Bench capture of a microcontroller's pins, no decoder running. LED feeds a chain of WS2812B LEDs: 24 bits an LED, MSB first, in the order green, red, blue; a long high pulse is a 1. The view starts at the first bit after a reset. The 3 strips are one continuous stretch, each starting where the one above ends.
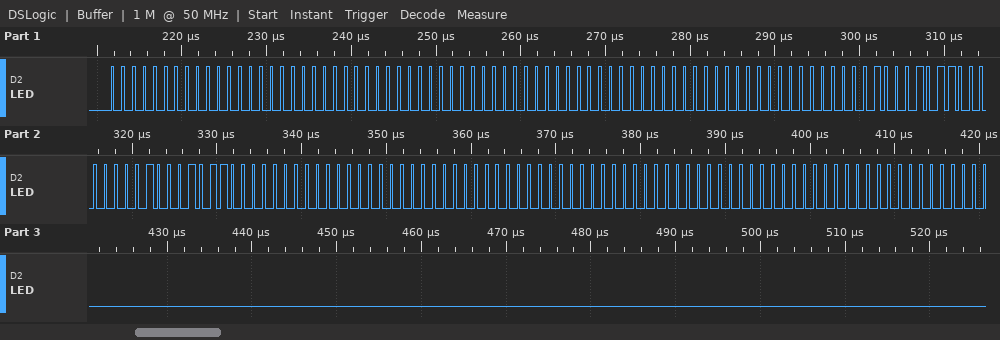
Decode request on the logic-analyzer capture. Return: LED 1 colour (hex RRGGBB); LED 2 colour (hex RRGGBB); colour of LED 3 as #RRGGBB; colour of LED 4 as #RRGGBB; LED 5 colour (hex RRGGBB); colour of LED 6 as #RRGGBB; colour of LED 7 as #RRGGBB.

#000000
#000000
#000000
#008B8B
#000000
#000000
#000000
